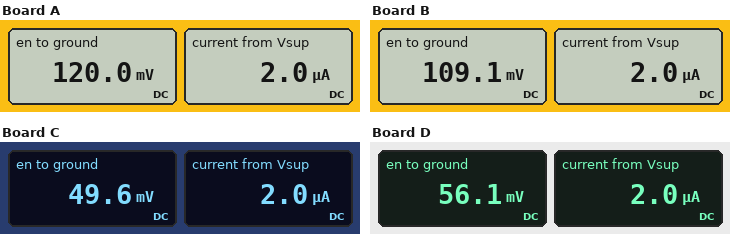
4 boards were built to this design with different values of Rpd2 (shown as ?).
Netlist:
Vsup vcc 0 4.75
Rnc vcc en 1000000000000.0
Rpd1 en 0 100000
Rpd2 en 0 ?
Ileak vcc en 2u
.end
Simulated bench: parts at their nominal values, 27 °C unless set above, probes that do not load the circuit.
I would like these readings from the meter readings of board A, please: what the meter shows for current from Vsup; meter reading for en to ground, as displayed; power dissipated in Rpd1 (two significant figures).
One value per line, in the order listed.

2.0 µA
120.0 mV
140 nW
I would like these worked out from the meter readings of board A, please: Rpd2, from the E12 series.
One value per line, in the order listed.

150 kΩ
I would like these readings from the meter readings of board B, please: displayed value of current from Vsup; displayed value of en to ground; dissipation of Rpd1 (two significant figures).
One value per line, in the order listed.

2.0 µA
109.1 mV
120 nW
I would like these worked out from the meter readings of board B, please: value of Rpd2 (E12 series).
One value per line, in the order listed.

120 kΩ
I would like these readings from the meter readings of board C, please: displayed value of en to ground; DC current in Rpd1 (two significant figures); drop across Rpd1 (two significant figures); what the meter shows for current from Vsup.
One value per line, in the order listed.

49.6 mV
500 nA
50 mV
2.0 µA
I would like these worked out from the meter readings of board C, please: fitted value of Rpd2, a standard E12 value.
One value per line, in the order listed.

33 kΩ
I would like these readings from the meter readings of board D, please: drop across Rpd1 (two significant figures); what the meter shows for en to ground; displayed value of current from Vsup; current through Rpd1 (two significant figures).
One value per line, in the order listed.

56 mV
56.1 mV
2.0 µA
560 nA
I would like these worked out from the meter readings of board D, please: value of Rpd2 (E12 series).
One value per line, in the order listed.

39 kΩ
